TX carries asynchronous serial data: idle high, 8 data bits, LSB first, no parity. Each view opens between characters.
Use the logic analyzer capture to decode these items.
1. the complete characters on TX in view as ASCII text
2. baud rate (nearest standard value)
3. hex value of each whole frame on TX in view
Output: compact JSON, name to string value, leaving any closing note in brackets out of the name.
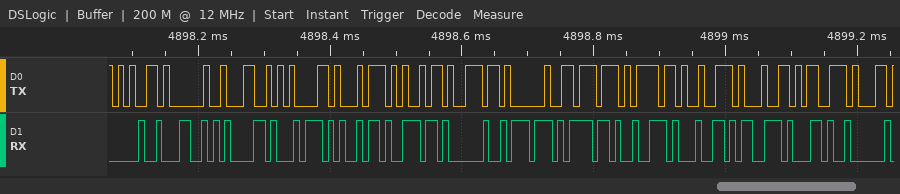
{"the complete characters on TX in view as ASCII text": "\"e Latin words\"", "baud rate": "115200 baud", "hex value of each whole frame on TX in view": "65, 20, 4C, 61, 74, 69, 6E, 20, 77, 6F, 72, 64, 73"}
